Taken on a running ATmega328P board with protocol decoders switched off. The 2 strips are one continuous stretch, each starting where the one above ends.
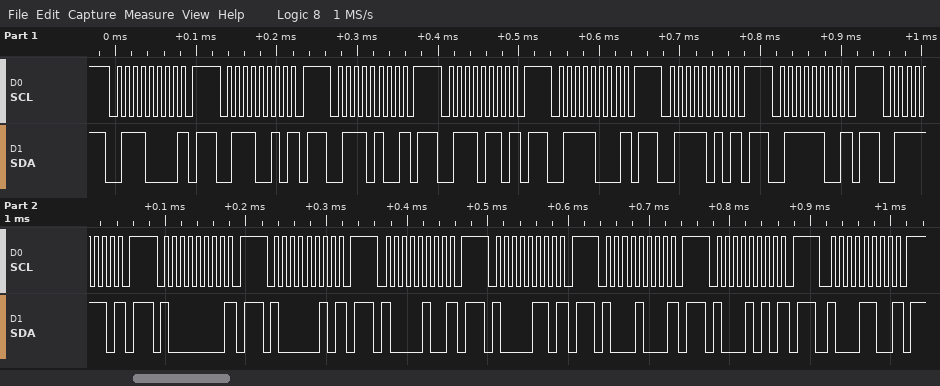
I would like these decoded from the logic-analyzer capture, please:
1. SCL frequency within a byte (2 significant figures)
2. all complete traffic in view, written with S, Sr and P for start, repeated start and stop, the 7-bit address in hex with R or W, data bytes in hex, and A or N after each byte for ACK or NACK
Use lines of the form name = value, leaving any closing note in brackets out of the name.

SCL frequency within a byte = 100 kHz
all complete traffic in view, written with S, Sr and P for start, repeated start and stop, the 7-bit address in hex with R or W, data bytes in hex, and A or N after each byte for ACK or NACK = S 38W N P S 39W N P S 3AW N P S 3BW N P S 3CW N P S 3DW N P S 3EW N P S 3FW N P S 40W N P S 41W N P S 42W N P S 43W N P S 44W N P S 45W N P S 46W N P
